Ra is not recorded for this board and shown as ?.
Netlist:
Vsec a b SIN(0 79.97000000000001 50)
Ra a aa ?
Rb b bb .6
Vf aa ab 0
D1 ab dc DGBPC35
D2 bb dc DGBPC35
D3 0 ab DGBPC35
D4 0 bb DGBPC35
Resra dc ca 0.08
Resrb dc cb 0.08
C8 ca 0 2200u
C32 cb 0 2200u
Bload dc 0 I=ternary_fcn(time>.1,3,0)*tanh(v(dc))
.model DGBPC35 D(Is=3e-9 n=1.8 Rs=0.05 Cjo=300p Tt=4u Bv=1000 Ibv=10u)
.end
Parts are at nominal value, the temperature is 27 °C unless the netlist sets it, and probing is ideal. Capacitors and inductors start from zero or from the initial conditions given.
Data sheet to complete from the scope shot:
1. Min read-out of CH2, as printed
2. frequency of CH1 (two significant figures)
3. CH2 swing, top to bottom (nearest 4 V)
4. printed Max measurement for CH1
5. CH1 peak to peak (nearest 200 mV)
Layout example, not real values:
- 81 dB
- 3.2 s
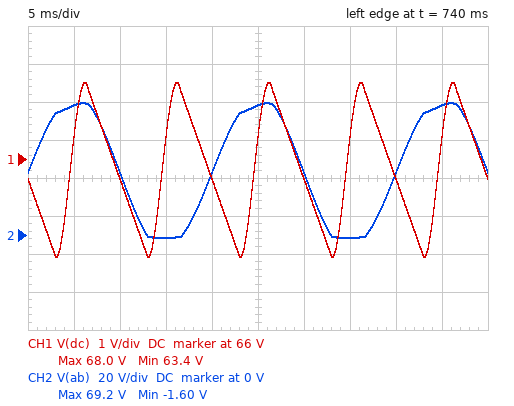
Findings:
- -1.60 V
- 100 Hz
- 72 V
- 68.0 V
- 4.6 V
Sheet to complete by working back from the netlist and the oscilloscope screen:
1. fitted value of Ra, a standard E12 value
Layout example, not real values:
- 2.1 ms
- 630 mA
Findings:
- 0.22 Ω
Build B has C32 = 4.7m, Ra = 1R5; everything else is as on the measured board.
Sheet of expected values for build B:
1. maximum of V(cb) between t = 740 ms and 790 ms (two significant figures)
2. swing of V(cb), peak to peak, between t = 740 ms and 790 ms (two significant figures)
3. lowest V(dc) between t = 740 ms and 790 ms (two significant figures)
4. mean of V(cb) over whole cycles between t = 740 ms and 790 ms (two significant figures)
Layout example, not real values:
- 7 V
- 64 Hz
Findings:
- 58 V
- 2.4 V
- 55 V
- 57 V
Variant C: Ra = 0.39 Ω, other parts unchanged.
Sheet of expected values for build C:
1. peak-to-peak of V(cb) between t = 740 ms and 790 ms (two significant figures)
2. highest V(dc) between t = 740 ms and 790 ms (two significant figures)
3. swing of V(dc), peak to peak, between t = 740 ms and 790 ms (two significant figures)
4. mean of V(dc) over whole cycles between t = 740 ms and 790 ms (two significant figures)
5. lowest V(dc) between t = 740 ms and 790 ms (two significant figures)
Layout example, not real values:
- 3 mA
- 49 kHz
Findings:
- 4.4 V
- 67 V
- 4.5 V
- 64 V
- 62 V
